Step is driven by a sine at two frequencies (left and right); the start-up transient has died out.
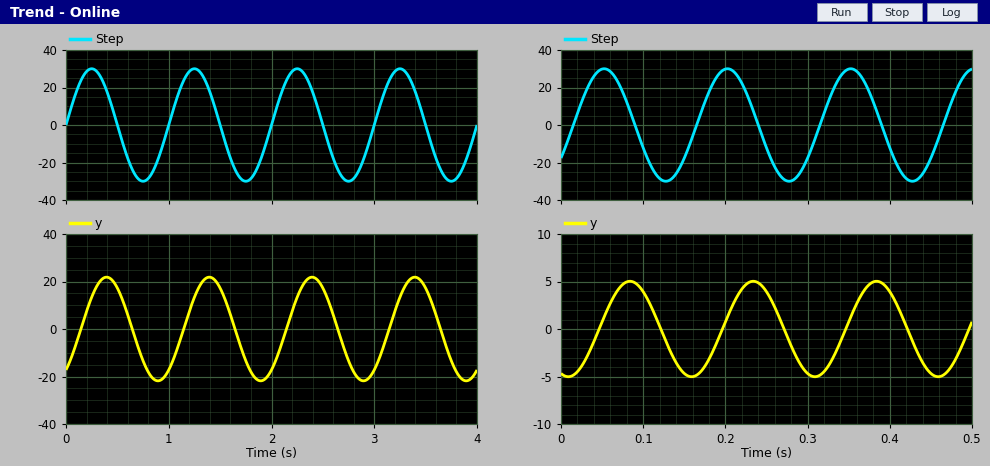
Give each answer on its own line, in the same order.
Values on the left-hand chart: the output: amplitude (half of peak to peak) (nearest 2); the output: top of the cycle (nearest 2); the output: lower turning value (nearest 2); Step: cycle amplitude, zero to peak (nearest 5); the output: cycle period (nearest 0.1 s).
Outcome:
22
22
-22
30
1.0 s
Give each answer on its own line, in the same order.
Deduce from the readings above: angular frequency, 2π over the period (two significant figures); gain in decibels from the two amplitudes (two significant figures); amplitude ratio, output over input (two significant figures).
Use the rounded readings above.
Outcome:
6.3 rad/s
-2.7 dB
0.73
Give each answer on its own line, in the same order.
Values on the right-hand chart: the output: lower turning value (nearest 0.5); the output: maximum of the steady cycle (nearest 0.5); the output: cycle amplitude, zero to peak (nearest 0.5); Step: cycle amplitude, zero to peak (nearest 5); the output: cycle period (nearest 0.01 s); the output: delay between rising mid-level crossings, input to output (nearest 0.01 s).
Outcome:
-5.0
5.0
5.0
30
0.15 s
0.03 s
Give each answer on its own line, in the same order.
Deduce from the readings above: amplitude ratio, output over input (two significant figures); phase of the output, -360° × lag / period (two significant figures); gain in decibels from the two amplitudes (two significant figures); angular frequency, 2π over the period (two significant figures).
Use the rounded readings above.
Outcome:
0.17
-72°
-16 dB
42 rad/s
